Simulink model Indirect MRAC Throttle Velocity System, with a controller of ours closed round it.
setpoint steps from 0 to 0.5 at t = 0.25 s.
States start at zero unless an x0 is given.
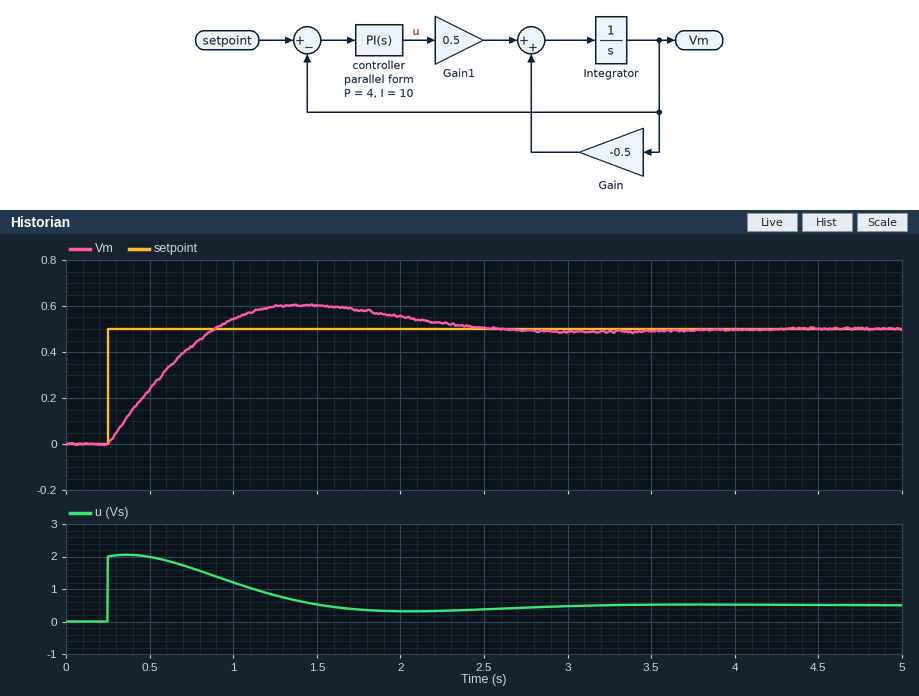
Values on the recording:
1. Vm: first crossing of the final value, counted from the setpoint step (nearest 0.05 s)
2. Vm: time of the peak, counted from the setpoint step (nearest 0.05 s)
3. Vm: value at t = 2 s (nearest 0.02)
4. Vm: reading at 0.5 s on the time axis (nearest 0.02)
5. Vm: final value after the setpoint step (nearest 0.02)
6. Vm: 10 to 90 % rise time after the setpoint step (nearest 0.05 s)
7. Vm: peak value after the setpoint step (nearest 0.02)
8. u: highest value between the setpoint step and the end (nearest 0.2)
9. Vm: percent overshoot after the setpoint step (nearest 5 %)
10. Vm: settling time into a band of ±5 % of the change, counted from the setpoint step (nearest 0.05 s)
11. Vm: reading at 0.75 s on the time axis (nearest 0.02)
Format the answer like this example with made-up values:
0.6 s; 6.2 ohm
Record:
0.65 s; 1.15 s; 0.56; 0.24; 0.50; 0.50 s; 0.60; 2.0; 20 %; 2.00 s; 0.42
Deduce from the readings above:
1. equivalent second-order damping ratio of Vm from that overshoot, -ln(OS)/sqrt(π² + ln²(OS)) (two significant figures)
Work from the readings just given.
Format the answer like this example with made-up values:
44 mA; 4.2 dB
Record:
0.46
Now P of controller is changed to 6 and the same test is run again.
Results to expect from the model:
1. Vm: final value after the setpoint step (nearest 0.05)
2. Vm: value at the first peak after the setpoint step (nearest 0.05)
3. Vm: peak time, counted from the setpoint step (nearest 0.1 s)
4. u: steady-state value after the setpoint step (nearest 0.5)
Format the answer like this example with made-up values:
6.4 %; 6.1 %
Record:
0.50; 0.55; 1.1 s; 0.5
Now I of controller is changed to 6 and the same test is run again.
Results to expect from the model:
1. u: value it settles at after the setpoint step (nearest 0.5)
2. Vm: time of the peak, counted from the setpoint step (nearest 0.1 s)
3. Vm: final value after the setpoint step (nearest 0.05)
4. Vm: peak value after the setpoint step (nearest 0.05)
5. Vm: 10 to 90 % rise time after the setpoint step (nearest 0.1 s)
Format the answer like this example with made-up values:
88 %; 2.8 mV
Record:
0.5; 1.5 s; 0.50; 0.55; 0.6 s
